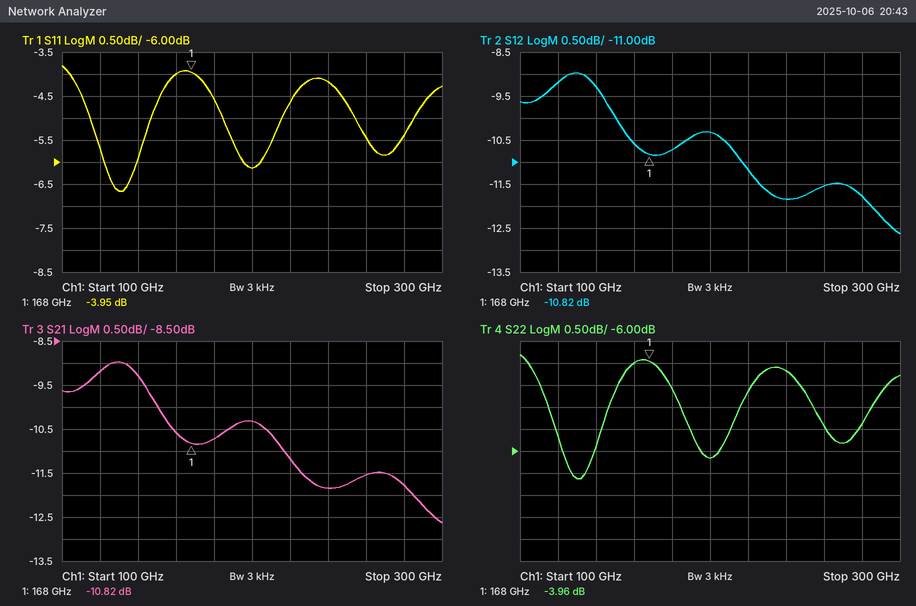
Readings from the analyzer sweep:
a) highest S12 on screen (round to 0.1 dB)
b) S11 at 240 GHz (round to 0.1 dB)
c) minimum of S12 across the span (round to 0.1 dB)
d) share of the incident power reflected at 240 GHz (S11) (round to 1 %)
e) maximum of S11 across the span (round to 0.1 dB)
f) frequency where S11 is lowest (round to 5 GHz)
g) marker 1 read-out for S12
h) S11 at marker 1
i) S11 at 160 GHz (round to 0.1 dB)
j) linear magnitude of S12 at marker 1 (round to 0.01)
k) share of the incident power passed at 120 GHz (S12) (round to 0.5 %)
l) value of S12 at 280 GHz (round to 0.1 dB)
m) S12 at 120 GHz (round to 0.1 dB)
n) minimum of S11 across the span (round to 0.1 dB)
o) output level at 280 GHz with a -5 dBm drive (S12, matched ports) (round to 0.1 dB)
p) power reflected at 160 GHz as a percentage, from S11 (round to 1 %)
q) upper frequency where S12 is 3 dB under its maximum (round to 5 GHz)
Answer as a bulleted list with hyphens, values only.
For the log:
- -9.0 dB
- -4.2 dB
- -12.6 dB
- 38 %
- -3.8 dB
- 130 GHz
- -10.82 dB
- -3.95 dB
- -4.0 dB
- 0.29
- 12.0 %
- -11.8 dB
- -9.2 dB
- -6.7 dB
- -16.8 dBm
- 40 %
- 285 GHz
